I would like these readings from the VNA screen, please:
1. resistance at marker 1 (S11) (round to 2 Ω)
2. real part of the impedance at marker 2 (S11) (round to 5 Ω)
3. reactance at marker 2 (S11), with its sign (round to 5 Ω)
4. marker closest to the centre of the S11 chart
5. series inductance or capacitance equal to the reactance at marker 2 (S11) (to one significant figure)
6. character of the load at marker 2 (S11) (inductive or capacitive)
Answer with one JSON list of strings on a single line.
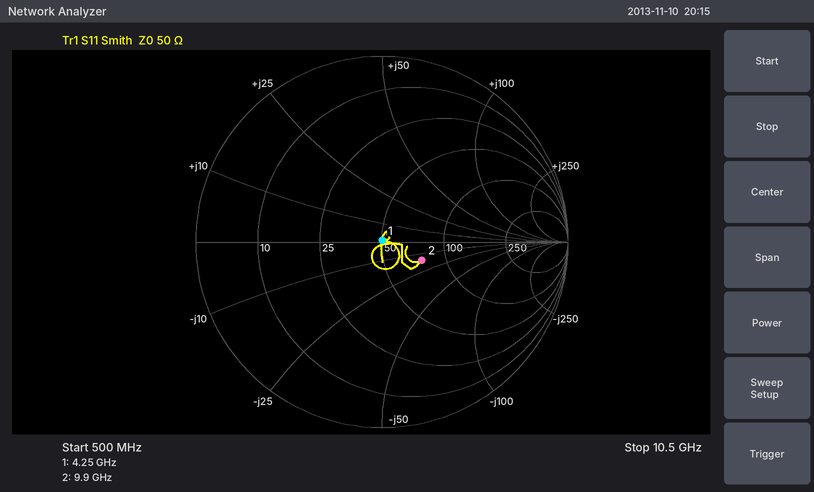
["50 Ω", "75 Ω", "-15 Ω", "marker 1", "1 pF", "capacitive"]
